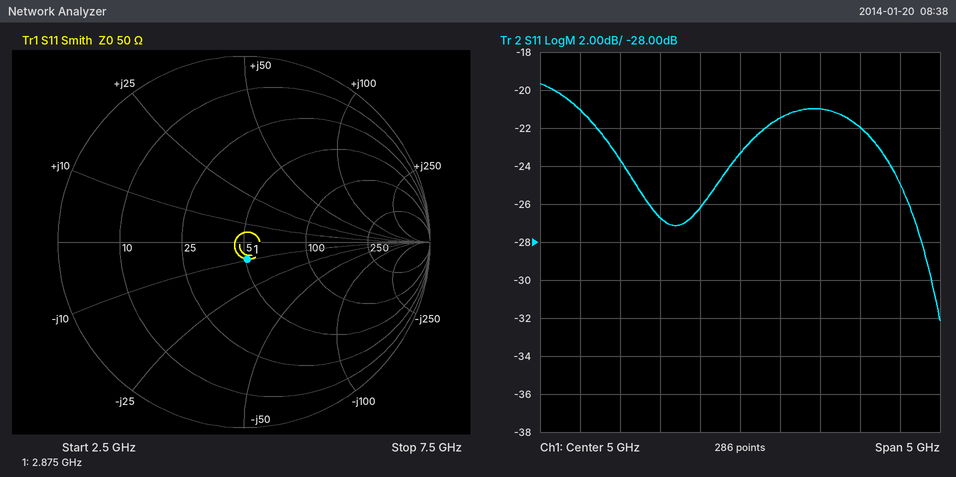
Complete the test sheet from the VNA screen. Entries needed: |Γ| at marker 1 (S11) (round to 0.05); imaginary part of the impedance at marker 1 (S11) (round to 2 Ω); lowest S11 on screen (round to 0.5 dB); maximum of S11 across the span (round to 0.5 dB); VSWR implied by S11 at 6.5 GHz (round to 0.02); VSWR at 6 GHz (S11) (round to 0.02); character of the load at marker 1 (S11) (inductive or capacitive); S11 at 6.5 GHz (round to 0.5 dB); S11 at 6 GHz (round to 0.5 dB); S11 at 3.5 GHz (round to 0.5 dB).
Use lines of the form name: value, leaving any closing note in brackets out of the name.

|Γ| at marker 1 (S11): 0.10
imaginary part of the impedance at marker 1 (S11): -10 Ω
lowest S11 on screen: -32.0 dB
maximum of S11 across the span: -19.5 dB
VSWR implied by S11 at 6.5 GHz: 1.18
VSWR at 6 GHz (S11): 1.20
character of the load at marker 1 (S11): capacitive
S11 at 6.5 GHz: -22.0 dB
S11 at 6 GHz: -21.0 dB
S11 at 3.5 GHz: -23.5 dB
